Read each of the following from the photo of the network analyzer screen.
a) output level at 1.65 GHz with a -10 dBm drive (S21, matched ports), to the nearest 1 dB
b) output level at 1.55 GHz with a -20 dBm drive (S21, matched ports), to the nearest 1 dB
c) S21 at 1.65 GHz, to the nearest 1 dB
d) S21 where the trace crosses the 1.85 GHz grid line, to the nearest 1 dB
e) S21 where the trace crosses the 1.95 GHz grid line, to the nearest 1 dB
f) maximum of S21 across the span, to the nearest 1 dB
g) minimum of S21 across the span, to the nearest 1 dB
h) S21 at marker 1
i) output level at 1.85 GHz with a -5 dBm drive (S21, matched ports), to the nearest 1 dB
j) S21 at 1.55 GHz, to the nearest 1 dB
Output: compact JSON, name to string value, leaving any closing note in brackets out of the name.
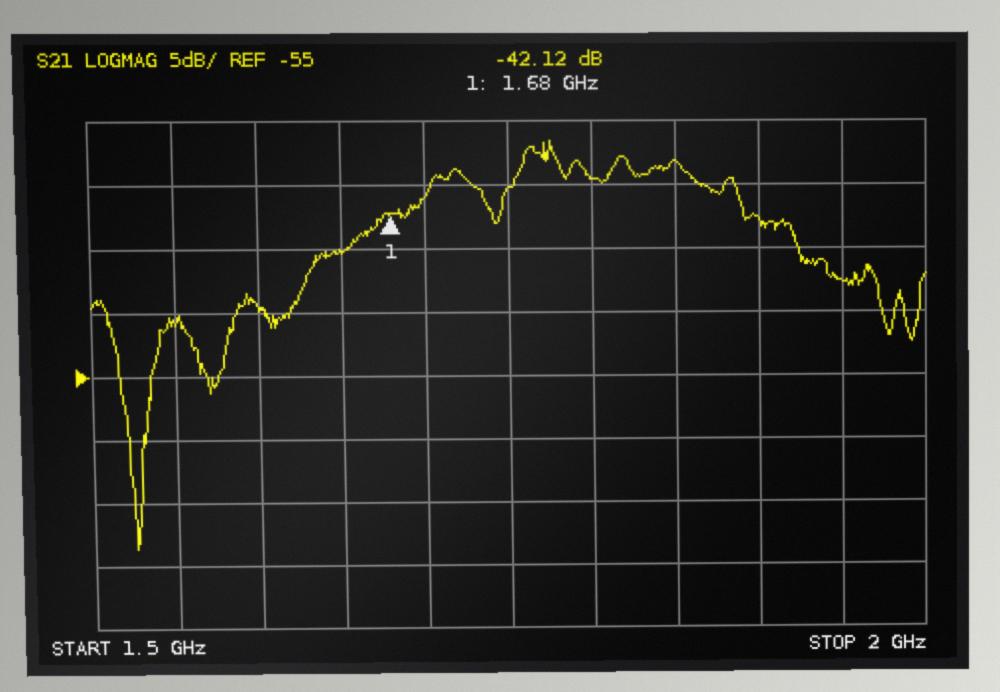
{"output level at 1.65 GHz with a -10 dBm drive (S21, matched ports), to the nearest 1 dB": "-55 dBm", "output level at 1.55 GHz with a -20 dBm drive (S21, matched ports), to the nearest 1 dB": "-71 dBm", "S21 at 1.65 GHz, to the nearest 1 dB": "-45 dB", "S21 where the trace crosses the 1.85 GHz grid line, to the nearest 1 dB": "-38 dB", "S21 where the trace crosses the 1.95 GHz grid line, to the nearest 1 dB": "-48 dB", "maximum of S21 across the span, to the nearest 1 dB": "-37 dB", "minimum of S21 across the span, to the nearest 1 dB": "-69 dB", "S21 at marker 1": "-42.12 dB", "output level at 1.85 GHz with a -5 dBm drive (S21, matched ports), to the nearest 1 dB": "-43 dBm", "S21 at 1.55 GHz, to the nearest 1 dB": "-51 dB"}
